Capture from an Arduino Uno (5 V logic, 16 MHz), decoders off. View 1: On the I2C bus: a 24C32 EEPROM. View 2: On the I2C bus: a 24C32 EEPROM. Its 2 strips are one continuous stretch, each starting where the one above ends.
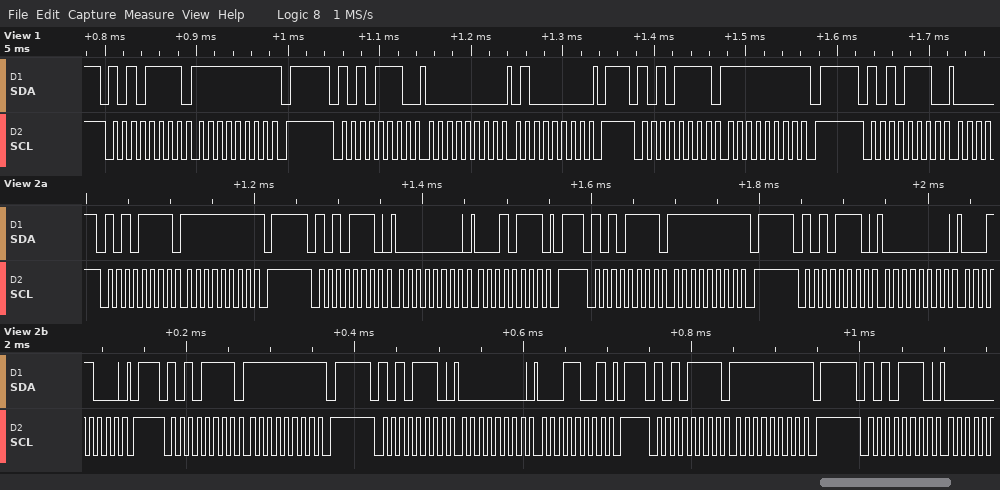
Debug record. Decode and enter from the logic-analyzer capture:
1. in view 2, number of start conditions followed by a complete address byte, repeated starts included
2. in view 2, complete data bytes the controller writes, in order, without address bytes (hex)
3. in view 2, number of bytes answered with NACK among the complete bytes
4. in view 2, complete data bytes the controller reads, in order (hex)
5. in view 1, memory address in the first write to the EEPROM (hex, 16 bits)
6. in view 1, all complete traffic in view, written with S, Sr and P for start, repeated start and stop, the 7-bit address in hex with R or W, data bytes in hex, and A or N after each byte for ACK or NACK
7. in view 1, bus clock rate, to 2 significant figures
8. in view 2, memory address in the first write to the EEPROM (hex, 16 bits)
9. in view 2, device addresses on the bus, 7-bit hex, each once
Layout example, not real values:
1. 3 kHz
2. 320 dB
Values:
1. 8
2. 00 17 00 18 00 19
3. 4
4. FF FF FF FF
5. 0x0040
6. S 57R A FF N P S 57W A 00 A 40 A P S 57R A FF N P S 57W A
7. 100 kHz
8. 0x0017
9. 0x57
